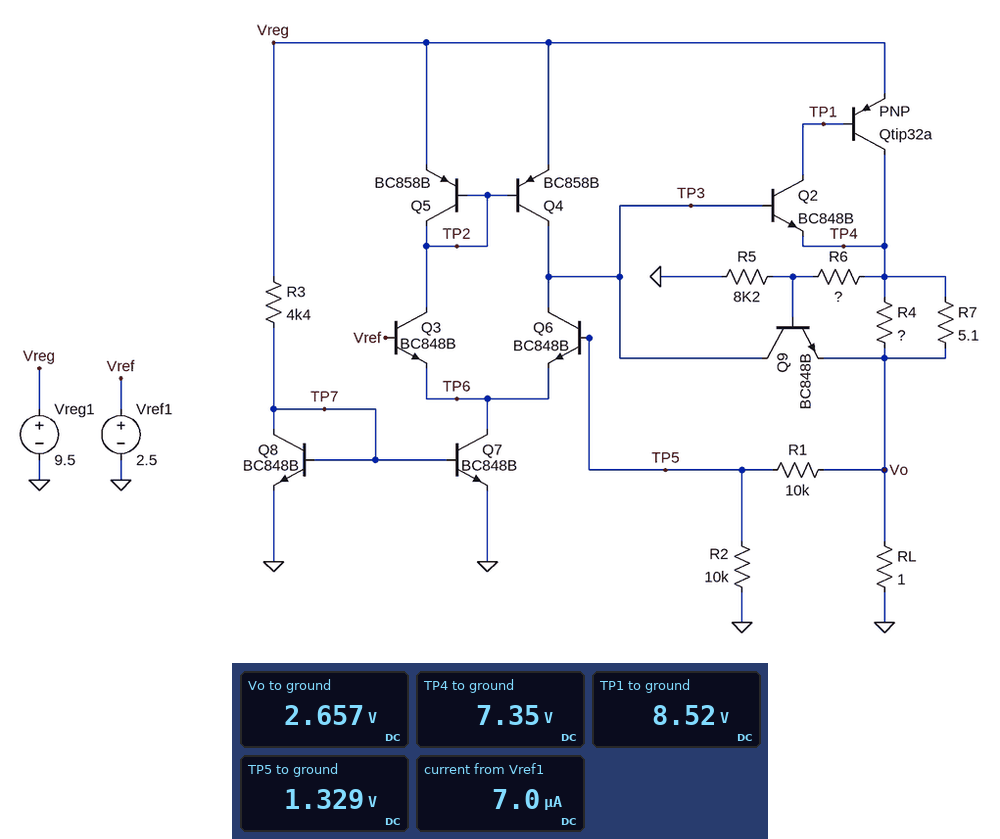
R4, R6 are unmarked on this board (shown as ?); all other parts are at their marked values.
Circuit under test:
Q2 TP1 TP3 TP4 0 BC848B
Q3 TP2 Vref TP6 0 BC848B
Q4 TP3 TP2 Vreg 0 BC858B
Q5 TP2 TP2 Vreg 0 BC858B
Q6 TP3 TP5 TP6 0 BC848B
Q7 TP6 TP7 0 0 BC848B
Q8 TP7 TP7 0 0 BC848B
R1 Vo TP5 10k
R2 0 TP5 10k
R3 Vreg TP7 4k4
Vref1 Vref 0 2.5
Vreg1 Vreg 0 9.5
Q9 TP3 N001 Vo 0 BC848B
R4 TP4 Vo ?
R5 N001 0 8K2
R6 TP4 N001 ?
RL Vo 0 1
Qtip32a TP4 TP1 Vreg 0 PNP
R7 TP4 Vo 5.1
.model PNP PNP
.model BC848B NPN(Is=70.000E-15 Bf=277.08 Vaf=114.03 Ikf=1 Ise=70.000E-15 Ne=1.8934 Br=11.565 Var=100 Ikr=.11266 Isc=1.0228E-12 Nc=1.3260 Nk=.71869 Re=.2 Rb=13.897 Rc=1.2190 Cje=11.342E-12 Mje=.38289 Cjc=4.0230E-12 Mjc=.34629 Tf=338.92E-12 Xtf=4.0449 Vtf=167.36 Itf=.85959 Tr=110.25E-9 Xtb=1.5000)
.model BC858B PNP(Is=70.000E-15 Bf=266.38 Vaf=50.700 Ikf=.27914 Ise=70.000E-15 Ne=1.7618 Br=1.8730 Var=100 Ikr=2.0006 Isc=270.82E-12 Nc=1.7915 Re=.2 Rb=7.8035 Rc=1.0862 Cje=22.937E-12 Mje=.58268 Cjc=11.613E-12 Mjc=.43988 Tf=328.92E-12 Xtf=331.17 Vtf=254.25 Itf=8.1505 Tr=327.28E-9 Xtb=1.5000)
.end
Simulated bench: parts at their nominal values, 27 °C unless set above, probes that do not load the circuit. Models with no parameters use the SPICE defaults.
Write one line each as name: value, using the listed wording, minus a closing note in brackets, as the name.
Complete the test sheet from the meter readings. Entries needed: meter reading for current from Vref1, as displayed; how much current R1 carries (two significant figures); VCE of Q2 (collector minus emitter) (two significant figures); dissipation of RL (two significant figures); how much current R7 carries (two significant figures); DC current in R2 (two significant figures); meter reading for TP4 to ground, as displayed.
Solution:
meter reading for current from Vref1, as displayed: 7.0 µA
how much current R1 carries: 130 µA
VCE of Q2 (collector minus emitter): 1.2 V
dissipation of RL: 7.1 W
how much current R7 carries: 920 mA
DC current in R2: 130 µA
meter reading for TP4 to ground, as displayed: 7.35 V
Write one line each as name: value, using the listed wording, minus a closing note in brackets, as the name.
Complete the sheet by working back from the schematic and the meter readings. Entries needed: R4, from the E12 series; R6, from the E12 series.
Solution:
R4, from the E12 series: 2.7 Ω
R6, from the E12 series: 10 kΩ
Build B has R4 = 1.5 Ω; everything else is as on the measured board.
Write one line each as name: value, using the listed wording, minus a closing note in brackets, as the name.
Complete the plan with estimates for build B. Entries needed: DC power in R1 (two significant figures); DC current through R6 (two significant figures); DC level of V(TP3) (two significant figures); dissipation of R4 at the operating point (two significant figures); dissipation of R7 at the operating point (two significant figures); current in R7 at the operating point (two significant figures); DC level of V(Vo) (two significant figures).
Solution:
DC power in R1: 380 µW
DC current through R6: 460 µA
DC level of V(TP3): 9.2 V
dissipation of R4 at the operating point: 14 W
dissipation of R7 at the operating point: 4.0 W
current in R7 at the operating point: 890 mA
DC level of V(Vo): 3.9 V
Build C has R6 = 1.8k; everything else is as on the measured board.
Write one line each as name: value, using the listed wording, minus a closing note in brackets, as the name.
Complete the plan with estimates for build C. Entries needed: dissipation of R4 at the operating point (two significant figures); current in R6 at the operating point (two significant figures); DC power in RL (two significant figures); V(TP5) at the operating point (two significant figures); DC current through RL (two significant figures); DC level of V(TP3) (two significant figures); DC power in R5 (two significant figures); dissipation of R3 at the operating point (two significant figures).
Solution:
dissipation of R4 at the operating point: 290 mW
current in R6 at the operating point: 150 µA
DC power in RL: 260 mW
V(TP5) at the operating point: 250 mV
DC current through RL: 510 mA
DC level of V(TP3): 2.0 V
DC power in R5: 160 µW
dissipation of R3 at the operating point: 18 mW
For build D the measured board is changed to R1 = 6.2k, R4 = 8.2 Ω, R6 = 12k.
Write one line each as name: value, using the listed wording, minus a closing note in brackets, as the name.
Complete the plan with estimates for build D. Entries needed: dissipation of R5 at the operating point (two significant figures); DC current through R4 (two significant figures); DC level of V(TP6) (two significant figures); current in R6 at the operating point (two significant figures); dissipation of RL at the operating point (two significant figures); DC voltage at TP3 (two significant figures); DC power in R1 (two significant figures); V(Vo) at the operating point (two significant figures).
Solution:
dissipation of R5 at the operating point: 310 µW
DC current through R4: 370 mA
DC level of V(TP6): 1.9 V
current in R6 at the operating point: 200 µA
dissipation of RL at the operating point: 950 mW
DC voltage at TP3: 4.7 V
DC power in R1: 22 µW
V(Vo) at the operating point: 970 mV
